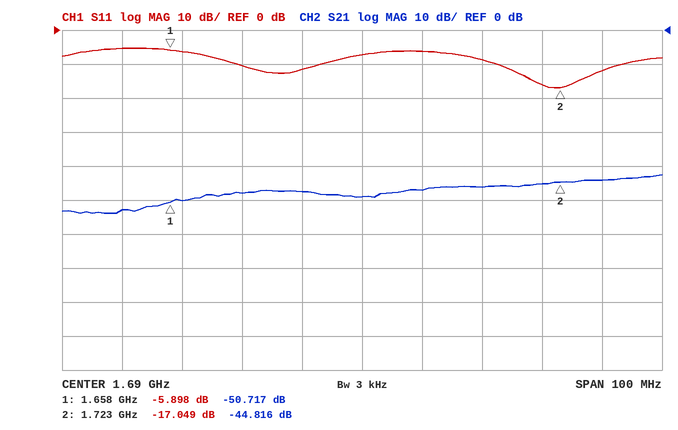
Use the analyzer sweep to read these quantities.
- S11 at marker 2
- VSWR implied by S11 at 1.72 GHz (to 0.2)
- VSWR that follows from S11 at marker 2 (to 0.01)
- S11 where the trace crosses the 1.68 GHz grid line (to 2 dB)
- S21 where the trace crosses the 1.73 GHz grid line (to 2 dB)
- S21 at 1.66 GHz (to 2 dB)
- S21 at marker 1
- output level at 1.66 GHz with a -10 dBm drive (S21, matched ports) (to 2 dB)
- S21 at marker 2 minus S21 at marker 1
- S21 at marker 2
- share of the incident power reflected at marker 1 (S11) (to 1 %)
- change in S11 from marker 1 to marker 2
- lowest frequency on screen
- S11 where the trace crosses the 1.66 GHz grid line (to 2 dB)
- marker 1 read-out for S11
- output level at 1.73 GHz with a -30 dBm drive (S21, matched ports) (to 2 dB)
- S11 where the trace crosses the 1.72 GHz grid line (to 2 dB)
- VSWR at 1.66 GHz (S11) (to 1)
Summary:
-17.049 dB
1.4
1.33
-12 dB
-44 dB
-50 dB
-50.717 dB
-60 dBm
5.901 dB
-44.816 dB
26 %
-11.151 dB
1.64 GHz
-6 dB
-5.898 dB
-74 dBm
-16 dB
3
